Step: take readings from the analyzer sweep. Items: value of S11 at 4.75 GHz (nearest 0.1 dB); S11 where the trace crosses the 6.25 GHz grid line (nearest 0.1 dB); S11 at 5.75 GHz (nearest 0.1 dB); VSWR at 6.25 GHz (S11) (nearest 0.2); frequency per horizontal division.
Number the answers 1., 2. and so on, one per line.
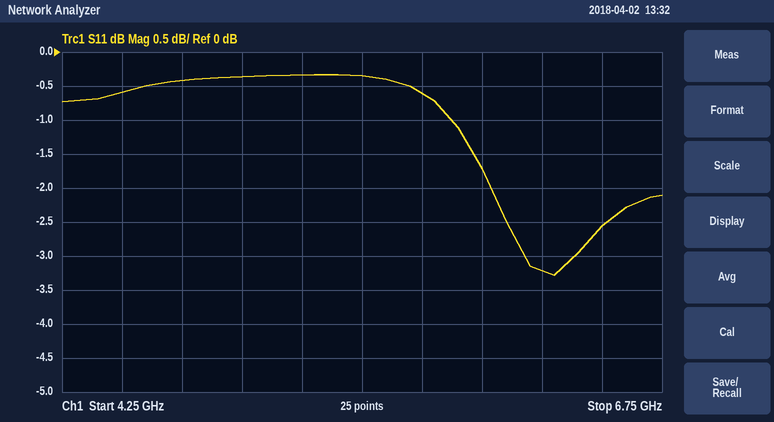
1. -0.4 dB
2. -3.2 dB
3. -0.6 dB
4. 5.4
5. 250 MHz
